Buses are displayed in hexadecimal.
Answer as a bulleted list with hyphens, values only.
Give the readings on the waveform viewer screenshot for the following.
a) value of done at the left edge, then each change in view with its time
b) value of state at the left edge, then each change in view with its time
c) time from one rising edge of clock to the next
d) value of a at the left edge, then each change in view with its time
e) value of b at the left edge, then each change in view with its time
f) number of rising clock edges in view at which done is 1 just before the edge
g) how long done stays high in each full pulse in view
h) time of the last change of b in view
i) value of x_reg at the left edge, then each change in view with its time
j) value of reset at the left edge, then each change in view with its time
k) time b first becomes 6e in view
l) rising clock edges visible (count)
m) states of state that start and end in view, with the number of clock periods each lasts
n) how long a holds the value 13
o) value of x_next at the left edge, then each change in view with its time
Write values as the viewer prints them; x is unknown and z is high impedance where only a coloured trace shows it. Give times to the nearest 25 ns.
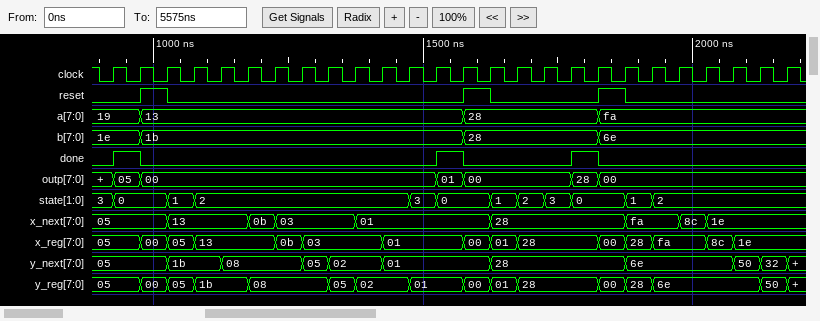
- 0, 1 at 925 ns, 0 at 975 ns, 1 at 1525 ns, 0 at 1575 ns, 1 at 1775 ns, 0 at 1825 ns
- 3, 0 at 925 ns, 1 at 1025 ns, 2 at 1075 ns, 3 at 1475 ns, 0 at 1525 ns, 1 at 1625 ns, 2 at 1675 ns, 3 at 1725 ns, 0 at 1775 ns, 1 at 1875 ns, 2 at 1925 ns
- 50 ns
- 19, 13 at 975 ns, 28 at 1575 ns, fa at 1825 ns
- 1e, 1b at 975 ns, 28 at 1575 ns, 6e at 1825 ns
- 3
- 50 ns, 50 ns, 50 ns
- 1825 ns
- 05, 00 at 975 ns, 05 at 1025 ns, 13 at 1075 ns, 0b at 1225 ns, 03 at 1275 ns, 01 at 1425 ns, 00 at 1575 ns, 01 at 1625 ns, 28 at 1675 ns, 00 at 1825 ns, 28 at 1875 ns, fa at 1925 ns, 8c at 2025 ns, 1e at 2075 ns
- 0, 1 at 975 ns, 0 at 1025 ns, 1 at 1575 ns, 0 at 1625 ns, 1 at 1825 ns, 0 at 1875 ns
- 1825 ns
- 26
- 0: 2, 1: 1, 2: 8, 3: 1, 0: 2, 1: 1, 2: 1, 3: 1, 0: 2, 1: 1
- 600 ns
- 05, 13 at 1025 ns, 0b at 1175 ns, 03 at 1225 ns, 01 at 1375 ns, 28 at 1625 ns, fa at 1875 ns, 8c at 1975 ns, 1e at 2025 ns
